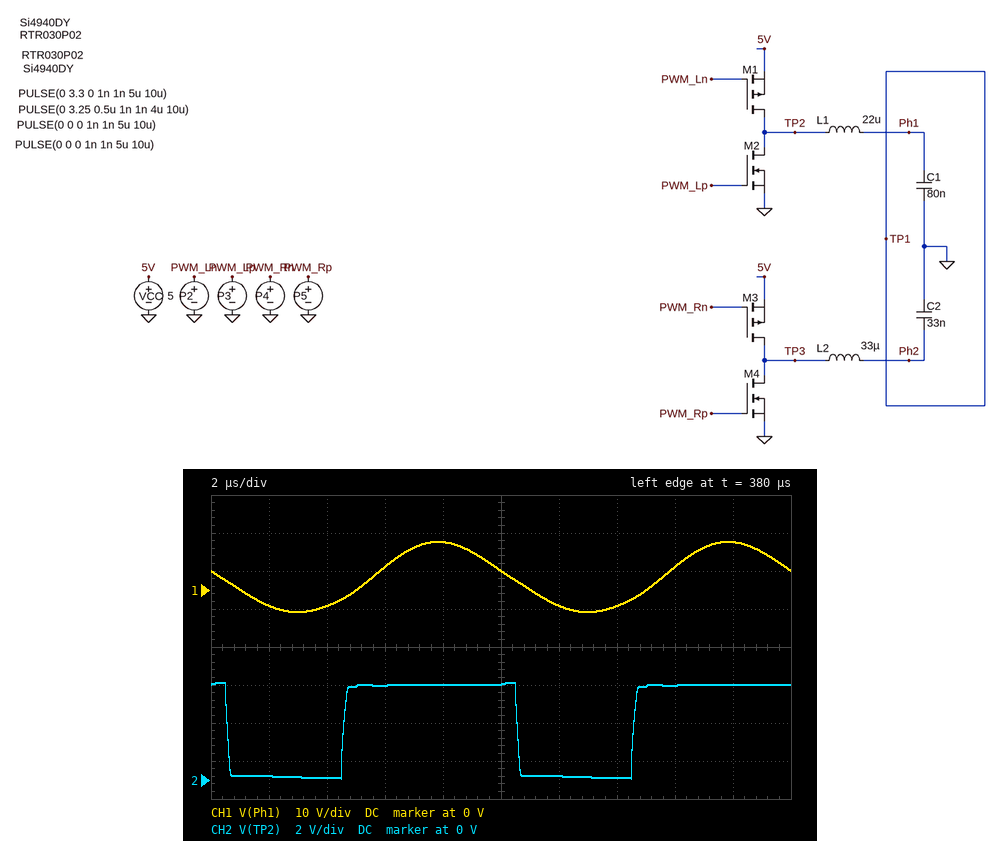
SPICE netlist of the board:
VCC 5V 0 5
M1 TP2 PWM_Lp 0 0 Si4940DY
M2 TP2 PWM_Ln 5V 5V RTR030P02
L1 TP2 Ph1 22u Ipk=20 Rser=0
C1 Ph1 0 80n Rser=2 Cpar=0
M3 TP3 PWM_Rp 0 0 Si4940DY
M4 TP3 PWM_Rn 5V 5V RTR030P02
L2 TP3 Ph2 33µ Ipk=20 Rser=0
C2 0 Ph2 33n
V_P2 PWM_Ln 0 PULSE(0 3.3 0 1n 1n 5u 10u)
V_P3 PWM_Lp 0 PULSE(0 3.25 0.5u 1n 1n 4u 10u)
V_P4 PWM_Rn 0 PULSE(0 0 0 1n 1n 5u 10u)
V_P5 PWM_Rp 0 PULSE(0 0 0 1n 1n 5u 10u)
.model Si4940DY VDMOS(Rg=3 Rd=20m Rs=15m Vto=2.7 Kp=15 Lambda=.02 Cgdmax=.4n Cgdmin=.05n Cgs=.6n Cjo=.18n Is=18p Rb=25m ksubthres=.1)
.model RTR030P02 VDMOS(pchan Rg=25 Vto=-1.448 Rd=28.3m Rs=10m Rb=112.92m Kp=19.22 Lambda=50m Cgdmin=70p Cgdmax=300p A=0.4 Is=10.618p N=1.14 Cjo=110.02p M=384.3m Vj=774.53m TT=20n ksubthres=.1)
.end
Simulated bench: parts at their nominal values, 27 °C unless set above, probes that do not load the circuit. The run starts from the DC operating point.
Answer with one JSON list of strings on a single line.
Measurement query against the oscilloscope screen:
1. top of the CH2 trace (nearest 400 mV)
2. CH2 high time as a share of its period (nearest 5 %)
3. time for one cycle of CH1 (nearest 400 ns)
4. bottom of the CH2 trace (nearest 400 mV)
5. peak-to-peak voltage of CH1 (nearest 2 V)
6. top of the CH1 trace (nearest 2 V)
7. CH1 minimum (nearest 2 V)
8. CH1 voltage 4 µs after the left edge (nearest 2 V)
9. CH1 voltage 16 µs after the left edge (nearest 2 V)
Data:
["5.2 V", "60 %", "10.0 µs", "0 V", "18 V", "12 V", "-6 V", "-4 V", "6 V"]
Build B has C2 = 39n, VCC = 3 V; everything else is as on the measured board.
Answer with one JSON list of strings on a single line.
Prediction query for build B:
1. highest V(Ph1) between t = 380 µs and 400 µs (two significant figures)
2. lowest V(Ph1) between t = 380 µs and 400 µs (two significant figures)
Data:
["7.8 V", "-4.2 V"]
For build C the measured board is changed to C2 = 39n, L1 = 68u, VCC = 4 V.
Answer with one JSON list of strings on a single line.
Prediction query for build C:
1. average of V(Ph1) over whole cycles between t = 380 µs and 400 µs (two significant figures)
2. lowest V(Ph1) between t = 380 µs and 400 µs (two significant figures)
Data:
["2.2 V", "120 mV"]
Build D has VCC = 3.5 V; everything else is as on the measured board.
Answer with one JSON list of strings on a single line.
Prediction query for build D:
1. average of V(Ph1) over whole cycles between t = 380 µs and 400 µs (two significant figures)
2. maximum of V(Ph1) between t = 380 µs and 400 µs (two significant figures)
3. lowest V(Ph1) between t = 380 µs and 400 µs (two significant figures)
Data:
["1.9 V", "9.1 V", "-4.9 V"]
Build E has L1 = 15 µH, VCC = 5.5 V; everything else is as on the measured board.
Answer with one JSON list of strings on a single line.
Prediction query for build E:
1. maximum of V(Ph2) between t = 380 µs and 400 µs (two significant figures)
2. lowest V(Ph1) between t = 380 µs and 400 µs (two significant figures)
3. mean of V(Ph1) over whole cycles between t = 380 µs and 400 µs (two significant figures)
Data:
["5.5 V", "5.1 V", "5.4 V"]
